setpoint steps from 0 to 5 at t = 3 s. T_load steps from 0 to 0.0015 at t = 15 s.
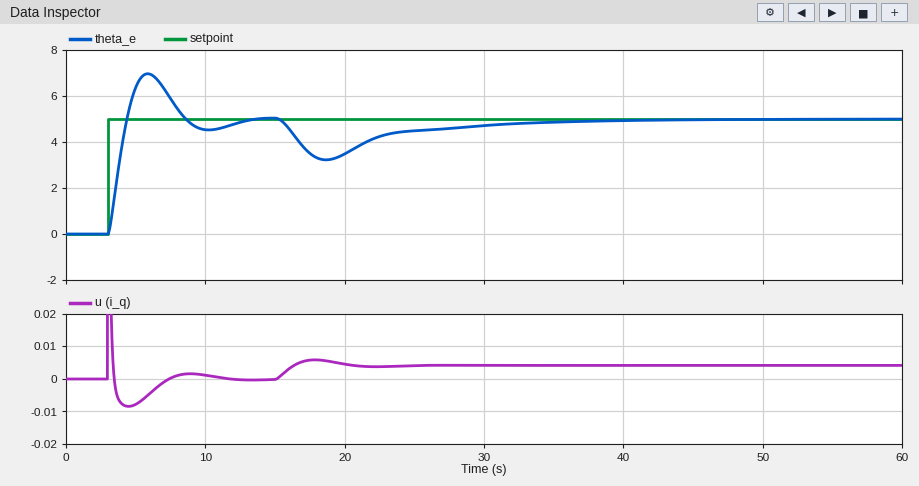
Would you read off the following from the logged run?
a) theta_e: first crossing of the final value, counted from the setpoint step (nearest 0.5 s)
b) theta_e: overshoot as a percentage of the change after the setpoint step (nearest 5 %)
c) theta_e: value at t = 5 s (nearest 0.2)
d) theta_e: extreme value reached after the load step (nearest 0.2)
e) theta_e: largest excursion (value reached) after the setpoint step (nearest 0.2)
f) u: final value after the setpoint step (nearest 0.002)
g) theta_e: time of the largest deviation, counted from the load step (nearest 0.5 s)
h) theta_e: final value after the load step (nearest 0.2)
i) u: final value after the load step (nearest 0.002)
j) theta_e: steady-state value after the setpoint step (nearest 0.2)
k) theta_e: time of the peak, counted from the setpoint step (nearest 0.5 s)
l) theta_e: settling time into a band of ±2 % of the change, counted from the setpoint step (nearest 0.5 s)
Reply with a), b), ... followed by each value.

a) 1.5 s
b) 40 %
c) 6.4
d) 3.2
e) 7.0
f) 0.000
g) 3.5 s
h) 5.0
i) 0.004
j) 5.0
k) 3.0 s
l) 10.0 s
